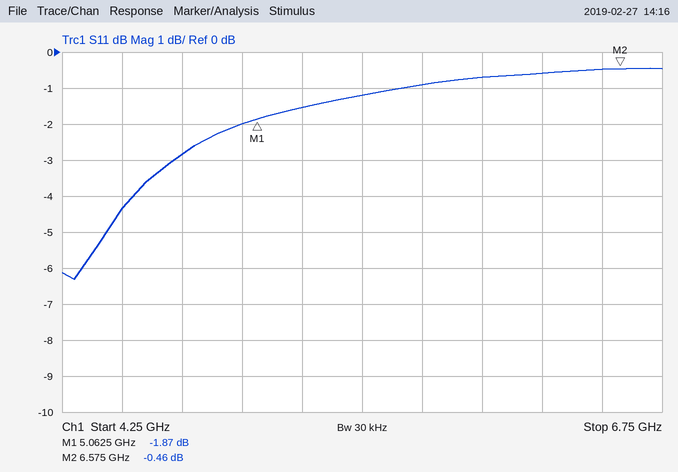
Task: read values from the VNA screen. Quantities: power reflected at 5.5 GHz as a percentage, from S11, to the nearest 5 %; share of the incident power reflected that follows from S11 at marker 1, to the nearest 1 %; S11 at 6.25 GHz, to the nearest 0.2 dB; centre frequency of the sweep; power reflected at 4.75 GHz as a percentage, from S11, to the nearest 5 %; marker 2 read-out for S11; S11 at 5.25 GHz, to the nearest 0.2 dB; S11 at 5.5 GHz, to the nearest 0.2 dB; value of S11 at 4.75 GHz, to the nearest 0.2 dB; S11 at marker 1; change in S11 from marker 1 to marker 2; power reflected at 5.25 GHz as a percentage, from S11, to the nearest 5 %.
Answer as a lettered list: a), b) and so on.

a) 75 %
b) 65 %
c) -0.6 dB
d) 5.5 GHz
e) 50 %
f) -0.46 dB
g) -1.6 dB
h) -1.2 dB
i) -2.8 dB
j) -1.87 dB
k) 1.41 dB
l) 70 %
